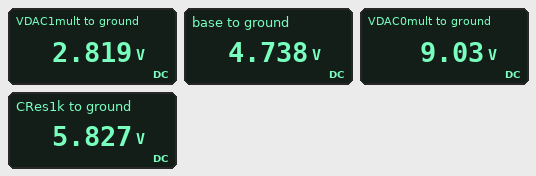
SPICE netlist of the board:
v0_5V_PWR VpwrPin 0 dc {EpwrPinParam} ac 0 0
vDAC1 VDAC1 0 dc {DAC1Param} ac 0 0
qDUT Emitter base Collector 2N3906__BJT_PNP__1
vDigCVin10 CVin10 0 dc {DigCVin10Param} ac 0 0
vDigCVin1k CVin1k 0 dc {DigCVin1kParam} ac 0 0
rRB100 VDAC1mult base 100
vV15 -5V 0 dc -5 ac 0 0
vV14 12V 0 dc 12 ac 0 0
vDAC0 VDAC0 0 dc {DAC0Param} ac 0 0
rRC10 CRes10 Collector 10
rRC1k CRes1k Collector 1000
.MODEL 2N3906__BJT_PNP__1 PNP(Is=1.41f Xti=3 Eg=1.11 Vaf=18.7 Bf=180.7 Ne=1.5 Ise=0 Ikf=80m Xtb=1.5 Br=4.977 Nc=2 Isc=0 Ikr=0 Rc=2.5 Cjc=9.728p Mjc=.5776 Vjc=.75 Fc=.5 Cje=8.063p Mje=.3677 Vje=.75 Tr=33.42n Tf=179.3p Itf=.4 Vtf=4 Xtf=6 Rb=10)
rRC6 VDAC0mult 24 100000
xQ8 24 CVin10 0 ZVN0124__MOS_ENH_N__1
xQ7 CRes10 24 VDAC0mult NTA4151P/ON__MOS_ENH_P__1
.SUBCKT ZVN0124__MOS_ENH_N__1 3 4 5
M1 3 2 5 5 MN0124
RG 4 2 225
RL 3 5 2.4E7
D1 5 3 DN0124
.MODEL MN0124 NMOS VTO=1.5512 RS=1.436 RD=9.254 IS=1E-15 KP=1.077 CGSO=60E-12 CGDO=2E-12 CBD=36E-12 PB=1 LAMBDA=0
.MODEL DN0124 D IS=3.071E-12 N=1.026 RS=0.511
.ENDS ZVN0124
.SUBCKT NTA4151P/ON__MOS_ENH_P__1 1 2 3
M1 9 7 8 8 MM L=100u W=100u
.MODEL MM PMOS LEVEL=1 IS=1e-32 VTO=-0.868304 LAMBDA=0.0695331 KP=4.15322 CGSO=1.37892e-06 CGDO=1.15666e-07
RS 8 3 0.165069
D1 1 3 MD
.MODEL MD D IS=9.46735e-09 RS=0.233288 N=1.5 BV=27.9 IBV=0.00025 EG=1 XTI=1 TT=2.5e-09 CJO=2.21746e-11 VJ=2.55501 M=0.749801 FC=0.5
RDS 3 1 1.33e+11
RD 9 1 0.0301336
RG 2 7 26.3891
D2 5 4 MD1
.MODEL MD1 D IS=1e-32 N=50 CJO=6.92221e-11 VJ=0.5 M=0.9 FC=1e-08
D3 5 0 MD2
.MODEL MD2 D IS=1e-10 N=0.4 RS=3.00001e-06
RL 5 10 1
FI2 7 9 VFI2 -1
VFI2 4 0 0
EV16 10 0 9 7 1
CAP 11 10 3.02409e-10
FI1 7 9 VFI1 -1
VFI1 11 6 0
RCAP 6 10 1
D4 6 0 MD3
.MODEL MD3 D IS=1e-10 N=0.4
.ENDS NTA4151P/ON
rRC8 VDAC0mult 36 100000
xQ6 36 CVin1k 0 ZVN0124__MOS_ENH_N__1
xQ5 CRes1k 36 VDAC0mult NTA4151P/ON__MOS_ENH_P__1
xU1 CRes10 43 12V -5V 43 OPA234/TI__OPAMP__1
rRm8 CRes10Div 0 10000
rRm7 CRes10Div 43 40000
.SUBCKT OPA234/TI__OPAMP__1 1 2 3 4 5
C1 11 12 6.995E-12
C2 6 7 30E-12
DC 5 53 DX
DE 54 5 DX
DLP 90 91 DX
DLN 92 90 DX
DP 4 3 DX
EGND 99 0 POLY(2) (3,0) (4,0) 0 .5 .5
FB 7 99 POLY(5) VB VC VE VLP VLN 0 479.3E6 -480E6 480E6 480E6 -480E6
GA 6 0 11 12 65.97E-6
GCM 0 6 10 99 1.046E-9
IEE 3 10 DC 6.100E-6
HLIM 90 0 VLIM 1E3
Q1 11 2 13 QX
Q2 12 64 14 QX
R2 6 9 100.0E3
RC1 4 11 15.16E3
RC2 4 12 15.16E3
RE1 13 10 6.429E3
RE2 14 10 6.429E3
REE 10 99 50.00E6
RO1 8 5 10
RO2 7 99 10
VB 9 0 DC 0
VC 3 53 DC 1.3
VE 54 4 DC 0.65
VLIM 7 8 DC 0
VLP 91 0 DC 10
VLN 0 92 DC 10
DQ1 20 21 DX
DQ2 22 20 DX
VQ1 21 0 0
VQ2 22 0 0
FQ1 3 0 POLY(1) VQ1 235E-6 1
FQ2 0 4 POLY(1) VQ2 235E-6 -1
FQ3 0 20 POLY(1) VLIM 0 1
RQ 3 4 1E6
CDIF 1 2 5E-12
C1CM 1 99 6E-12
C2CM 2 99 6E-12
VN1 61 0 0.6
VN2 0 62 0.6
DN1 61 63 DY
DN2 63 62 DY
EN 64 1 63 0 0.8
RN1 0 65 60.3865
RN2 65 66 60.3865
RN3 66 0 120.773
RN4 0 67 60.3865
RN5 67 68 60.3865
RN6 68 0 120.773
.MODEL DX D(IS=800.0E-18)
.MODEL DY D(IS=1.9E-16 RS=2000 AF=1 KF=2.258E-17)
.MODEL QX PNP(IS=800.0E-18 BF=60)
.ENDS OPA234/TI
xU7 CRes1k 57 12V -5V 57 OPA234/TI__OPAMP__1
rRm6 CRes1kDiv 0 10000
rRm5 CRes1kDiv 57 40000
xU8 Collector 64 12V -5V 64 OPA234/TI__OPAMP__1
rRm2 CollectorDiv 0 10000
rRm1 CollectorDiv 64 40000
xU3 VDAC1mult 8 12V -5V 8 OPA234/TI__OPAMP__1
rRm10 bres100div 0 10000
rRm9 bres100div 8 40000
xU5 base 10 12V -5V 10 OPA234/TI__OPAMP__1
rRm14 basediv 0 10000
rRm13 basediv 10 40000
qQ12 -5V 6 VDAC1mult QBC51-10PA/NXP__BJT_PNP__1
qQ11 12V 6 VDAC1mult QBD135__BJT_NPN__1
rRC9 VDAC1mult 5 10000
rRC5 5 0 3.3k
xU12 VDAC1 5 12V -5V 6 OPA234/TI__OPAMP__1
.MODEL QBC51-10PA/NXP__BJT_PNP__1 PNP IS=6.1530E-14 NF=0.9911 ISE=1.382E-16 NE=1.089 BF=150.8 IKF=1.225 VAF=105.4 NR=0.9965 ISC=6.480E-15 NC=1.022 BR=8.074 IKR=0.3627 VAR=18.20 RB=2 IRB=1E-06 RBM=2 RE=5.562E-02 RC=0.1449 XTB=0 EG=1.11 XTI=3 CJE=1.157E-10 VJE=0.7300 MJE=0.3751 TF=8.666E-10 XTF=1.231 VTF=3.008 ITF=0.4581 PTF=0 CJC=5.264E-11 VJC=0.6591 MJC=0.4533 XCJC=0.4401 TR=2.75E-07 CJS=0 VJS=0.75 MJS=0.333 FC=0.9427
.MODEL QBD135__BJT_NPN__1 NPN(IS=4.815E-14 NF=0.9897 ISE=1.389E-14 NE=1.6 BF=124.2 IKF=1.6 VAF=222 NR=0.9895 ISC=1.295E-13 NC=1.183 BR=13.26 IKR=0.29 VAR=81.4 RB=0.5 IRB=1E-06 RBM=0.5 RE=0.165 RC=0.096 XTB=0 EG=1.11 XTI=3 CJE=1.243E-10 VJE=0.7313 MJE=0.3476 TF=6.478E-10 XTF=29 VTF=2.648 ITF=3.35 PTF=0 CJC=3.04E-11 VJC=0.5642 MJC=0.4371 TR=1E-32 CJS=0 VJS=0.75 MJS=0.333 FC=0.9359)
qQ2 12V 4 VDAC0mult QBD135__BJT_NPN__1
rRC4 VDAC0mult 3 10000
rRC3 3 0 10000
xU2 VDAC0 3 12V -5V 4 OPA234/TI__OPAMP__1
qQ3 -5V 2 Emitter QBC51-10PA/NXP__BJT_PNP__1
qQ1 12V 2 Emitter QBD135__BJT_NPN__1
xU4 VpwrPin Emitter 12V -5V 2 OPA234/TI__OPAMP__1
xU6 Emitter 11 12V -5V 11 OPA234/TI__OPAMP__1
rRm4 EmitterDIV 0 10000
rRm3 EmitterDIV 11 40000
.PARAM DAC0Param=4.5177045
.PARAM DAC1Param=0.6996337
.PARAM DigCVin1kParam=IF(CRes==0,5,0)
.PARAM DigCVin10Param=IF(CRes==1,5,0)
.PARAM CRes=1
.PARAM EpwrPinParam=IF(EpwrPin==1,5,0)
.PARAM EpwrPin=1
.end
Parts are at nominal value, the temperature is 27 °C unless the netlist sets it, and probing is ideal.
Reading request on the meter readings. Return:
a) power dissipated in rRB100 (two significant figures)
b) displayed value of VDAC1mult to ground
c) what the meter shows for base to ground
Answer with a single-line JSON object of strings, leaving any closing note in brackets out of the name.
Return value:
{"power dissipated in rRB100": "37 mW", "displayed value of VDAC1mult to ground": "2.819 V", "what the meter shows for base to ground": "4.738 V"}
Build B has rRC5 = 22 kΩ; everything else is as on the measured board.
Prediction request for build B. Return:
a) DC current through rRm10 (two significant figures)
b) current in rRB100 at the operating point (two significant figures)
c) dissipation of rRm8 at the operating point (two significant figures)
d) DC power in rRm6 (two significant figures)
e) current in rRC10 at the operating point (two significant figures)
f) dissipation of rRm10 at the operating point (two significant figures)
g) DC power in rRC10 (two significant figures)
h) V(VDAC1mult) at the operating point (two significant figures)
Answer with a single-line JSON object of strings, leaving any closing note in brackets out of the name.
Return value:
{"DC current through rRm10": "20 µA", "current in rRB100 at the operating point": "35 mA", "dissipation of rRm8 at the operating point": "320 µW", "DC power in rRm6": "130 µW", "current in rRC10 at the operating point": "320 mA", "dissipation of rRm10 at the operating point": "4.1 µW", "DC power in rRC10": "1.0 W", "V(VDAC1mult) at the operating point": "1.0 V"}
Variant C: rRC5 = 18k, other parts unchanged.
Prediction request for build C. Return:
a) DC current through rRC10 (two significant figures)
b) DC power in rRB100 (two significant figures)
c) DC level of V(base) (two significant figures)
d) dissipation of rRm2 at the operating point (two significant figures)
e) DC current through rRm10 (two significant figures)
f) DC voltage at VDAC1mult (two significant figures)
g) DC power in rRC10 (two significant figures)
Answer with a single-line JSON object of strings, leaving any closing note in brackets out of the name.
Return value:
{"DC current through rRC10": "320 mA", "DC power in rRB100": "120 mW", "DC level of V(base)": "4.5 V", "dissipation of rRm2 at the operating point": "130 µW", "DC current through rRm10": "22 µA", "DC voltage at VDAC1mult": "1.1 V", "DC power in rRC10": "1.0 W"}
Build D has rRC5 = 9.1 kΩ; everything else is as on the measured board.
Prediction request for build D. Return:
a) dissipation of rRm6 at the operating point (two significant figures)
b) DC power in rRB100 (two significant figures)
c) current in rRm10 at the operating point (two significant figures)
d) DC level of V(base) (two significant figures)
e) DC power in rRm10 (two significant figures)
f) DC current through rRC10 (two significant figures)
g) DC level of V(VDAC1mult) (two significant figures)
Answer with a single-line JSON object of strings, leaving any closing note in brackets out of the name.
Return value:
{"dissipation of rRm6 at the operating point": "130 µW", "DC power in rRB100": "97 mW", "current in rRm10 at the operating point": "29 µA", "DC level of V(base)": "4.6 V", "DC power in rRm10": "8.6 µW", "DC current through rRC10": "320 mA", "DC level of V(VDAC1mult)": "1.5 V"}
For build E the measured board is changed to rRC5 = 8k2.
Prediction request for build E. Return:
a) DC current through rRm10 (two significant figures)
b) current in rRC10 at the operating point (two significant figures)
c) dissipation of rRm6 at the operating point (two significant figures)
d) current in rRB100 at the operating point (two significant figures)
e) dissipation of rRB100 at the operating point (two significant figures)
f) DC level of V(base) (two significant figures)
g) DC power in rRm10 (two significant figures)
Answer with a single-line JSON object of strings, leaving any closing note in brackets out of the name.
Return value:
{"DC current through rRm10": "31 µA", "current in rRC10 at the operating point": "320 mA", "dissipation of rRm6 at the operating point": "130 µW", "current in rRB100 at the operating point": "30 mA", "dissipation of rRB100 at the operating point": "92 mW", "DC level of V(base)": "4.6 V", "DC power in rRm10": "9.6 µW"}
